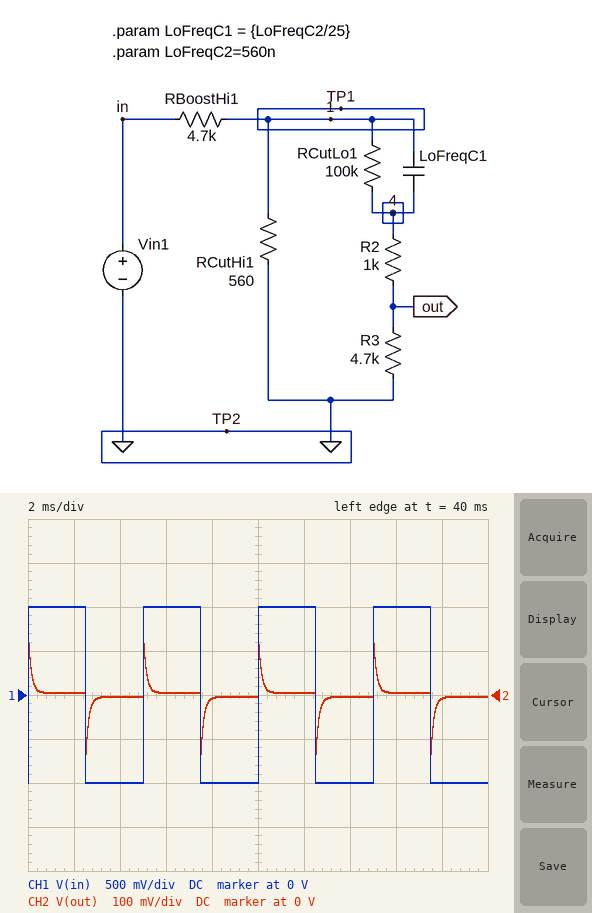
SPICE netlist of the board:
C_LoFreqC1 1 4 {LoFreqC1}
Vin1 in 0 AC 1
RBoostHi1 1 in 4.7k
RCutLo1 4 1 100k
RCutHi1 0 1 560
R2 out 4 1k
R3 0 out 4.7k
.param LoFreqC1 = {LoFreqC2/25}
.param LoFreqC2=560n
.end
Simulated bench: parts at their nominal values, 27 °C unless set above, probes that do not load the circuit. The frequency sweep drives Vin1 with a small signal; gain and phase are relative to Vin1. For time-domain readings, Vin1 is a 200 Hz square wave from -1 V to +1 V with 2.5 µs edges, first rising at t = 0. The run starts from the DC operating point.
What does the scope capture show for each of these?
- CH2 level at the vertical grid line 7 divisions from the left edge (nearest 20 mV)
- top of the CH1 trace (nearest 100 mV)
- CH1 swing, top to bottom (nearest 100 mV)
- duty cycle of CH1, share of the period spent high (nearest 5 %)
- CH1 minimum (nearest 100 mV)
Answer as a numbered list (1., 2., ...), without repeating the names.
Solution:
1. 0 V
2. 1.0 V
3. 2.0 V
4. 50 %
5. -1.0 V
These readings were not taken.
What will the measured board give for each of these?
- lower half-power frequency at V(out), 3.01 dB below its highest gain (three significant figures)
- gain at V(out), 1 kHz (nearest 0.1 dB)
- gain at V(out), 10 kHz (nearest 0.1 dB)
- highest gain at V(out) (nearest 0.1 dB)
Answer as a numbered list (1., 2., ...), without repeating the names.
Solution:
1. 1.21 kHz
2. -25.8 dB
3. -21.9 dB
4. -21.9 dB
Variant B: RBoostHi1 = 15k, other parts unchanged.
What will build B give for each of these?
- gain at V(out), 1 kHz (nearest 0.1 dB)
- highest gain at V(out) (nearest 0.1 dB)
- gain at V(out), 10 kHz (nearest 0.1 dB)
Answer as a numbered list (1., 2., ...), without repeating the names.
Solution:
1. -35.2 dB
2. -31.3 dB
3. -31.4 dB
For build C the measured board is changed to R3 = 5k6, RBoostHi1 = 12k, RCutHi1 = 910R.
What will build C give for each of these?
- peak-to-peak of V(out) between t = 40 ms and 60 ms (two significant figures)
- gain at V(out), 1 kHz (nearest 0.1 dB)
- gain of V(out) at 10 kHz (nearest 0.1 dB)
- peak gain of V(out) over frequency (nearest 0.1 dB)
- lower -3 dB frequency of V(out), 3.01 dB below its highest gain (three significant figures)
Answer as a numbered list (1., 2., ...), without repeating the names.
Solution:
1. 200 mV
2. -28.6 dB
3. -25.6 dB
4. -25.5 dB
5. 1.02 kHz
